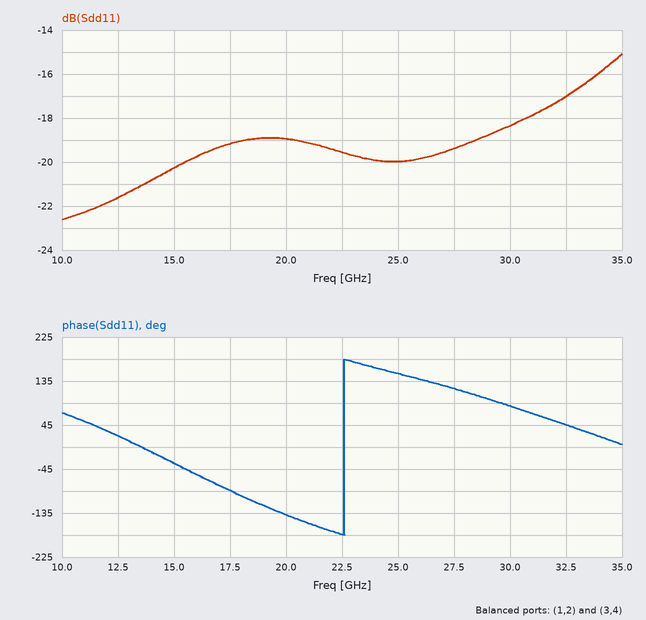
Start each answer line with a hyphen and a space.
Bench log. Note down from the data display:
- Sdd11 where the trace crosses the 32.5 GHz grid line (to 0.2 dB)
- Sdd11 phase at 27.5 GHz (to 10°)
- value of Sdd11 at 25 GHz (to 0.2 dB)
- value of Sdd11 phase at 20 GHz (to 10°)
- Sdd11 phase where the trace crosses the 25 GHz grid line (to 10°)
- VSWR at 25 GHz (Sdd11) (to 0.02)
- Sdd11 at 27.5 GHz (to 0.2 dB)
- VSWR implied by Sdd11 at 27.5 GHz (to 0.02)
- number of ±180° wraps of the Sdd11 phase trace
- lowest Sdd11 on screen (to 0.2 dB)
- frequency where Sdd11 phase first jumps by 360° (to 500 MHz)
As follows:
- -17.0 dB
- 120°
- -20.0 dB
- -140°
- 150°
- 1.22
- -19.4 dB
- 1.24
- 1
- -22.6 dB
- 22.5 GHz
